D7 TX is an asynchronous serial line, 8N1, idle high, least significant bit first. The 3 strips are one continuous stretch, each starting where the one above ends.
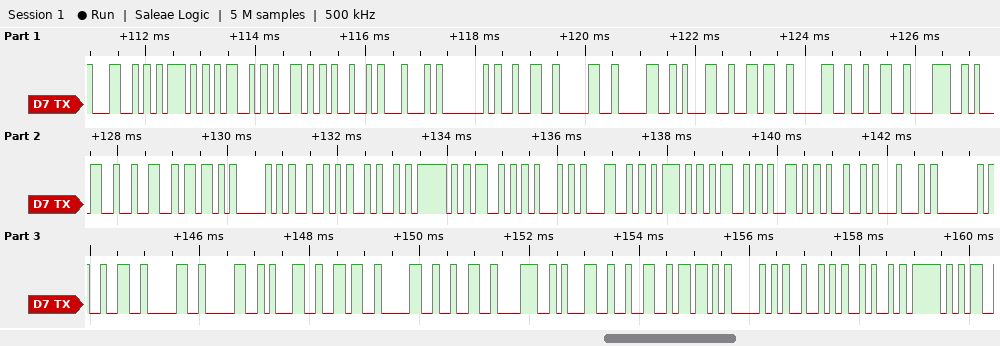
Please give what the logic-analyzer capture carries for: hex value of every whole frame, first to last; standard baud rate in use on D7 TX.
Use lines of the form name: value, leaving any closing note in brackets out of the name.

hex value of every whole frame, first to last: 4C 5D 4D 59 49 44 40 32 30 30 31 36 30 32 38 31 32 5B 50 52 4A 5F 53 51 4C 5D 4D 59 49 44 40 32 30 30 31 36 30 32 38 31 32 5B 50 52 4A 5F
standard baud rate in use on D7 TX: 9600 baud
